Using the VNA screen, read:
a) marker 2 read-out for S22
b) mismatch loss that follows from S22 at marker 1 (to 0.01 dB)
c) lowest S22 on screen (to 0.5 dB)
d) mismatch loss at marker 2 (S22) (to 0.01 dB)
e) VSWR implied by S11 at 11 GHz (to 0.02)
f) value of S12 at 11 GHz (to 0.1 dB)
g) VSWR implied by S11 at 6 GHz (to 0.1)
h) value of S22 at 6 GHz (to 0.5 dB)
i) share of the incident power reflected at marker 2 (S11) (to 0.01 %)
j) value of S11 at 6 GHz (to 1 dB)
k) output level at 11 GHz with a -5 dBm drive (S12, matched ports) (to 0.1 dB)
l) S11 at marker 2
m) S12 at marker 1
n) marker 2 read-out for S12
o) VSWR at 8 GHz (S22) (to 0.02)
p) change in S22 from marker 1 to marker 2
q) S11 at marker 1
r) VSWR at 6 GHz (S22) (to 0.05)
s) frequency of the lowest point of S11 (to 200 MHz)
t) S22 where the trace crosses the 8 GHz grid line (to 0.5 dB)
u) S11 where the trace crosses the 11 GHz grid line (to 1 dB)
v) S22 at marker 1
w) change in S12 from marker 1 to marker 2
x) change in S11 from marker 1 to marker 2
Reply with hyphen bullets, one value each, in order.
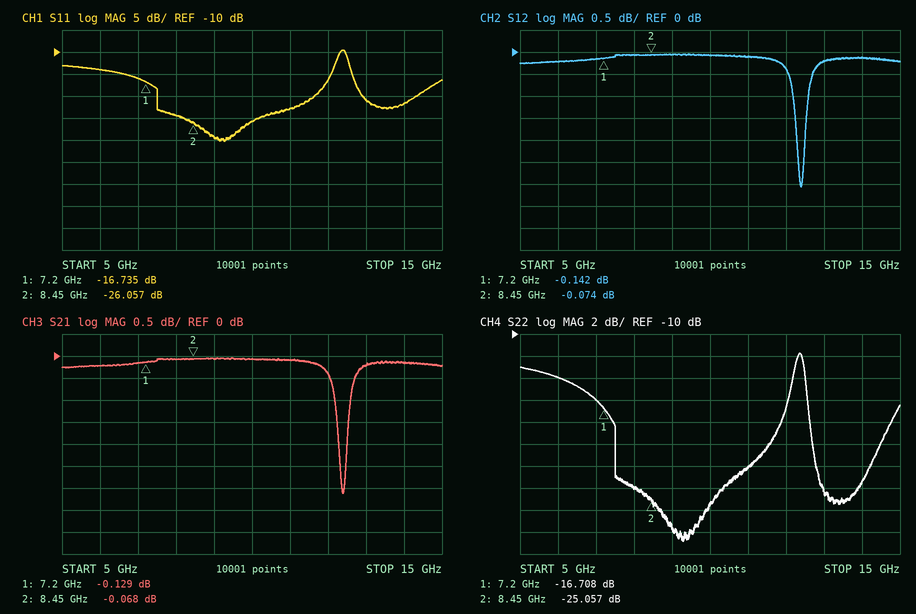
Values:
- -25.057 dB
- 0.09 dB
- -29.0 dB
- 0.01 dB
- 1.16
- -0.1 dB
- 1.5
- -14.0 dB
- 0.25 %
- -14 dB
- -5.1 dBm
- -26.057 dB
- -0.142 dB
- -0.074 dB
- 1.14
- -8.349 dB
- -16.735 dB
- 1.50
- 9.2 GHz
- -24.0 dB
- -23 dB
- -16.708 dB
- 0.068 dB
- -9.322 dB
